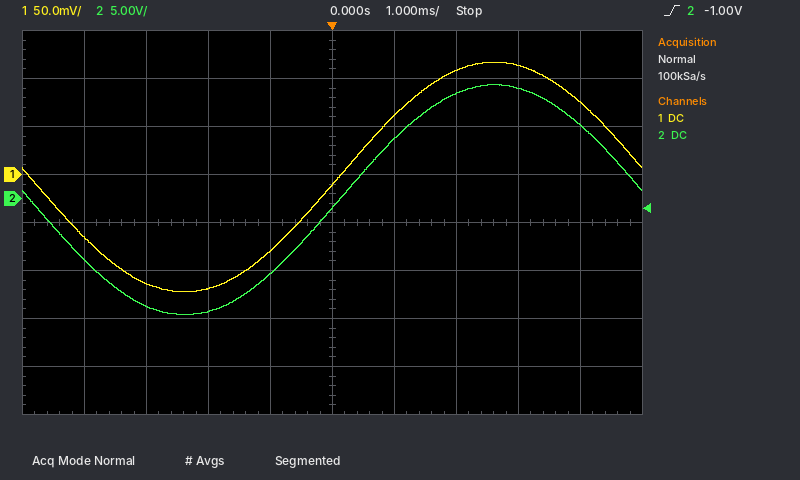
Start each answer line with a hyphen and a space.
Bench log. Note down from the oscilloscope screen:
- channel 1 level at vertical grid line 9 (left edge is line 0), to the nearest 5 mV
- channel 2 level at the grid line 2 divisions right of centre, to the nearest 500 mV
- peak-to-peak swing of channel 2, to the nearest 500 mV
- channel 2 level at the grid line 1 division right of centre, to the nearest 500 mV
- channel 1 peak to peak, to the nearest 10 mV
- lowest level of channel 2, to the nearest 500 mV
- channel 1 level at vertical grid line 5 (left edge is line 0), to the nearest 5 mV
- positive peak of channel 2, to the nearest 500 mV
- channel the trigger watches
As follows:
- 75 mV
- 11.0 V
- 24.0 V
- 6.0 V
- 240 mV
- -12.0 V
- -10 mV
- 12.0 V
- channel 2
